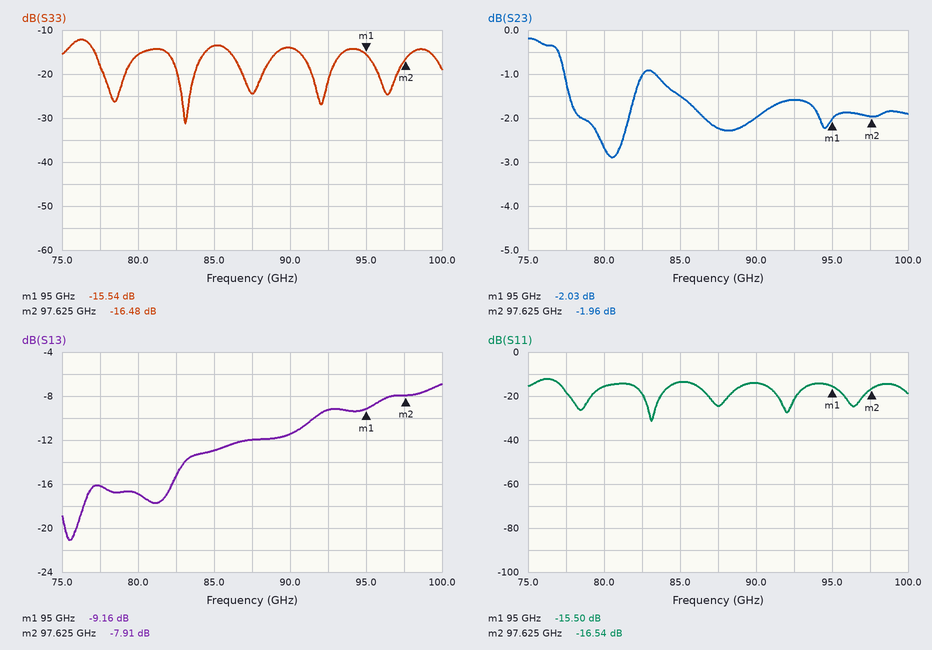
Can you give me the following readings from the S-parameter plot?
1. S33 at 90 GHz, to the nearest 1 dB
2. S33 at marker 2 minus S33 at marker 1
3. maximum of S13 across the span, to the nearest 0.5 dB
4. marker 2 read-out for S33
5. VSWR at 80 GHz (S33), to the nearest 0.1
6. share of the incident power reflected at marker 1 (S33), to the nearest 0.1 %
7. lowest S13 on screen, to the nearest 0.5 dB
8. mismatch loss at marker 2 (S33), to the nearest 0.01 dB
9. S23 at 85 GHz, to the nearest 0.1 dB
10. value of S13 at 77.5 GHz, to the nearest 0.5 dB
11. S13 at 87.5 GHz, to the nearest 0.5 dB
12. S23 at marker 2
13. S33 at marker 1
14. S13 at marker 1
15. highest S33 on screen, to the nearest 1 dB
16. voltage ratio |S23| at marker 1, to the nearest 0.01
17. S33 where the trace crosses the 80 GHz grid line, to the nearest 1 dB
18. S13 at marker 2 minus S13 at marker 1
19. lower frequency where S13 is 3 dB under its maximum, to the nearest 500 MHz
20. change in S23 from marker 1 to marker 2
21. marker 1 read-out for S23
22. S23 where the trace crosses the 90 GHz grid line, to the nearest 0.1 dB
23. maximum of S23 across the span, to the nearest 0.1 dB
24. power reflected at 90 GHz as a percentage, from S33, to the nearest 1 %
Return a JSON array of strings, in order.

["-14 dB", "-0.94 dB", "-7.0 dB", "-16.48 dB", "1.4", "2.8 %", "-21.0 dB", "0.10 dB", "-1.5 dB", "-16.0 dB", "-12.0 dB", "-1.96 dB", "-15.54 dB", "-9.16 dB", "-12 dB", "0.79", "-16 dB", "1.25 dB", "91.5 GHz", "0.07 dB", "-2.03 dB", "-2.0 dB", "-0.2 dB", "4 %"]
